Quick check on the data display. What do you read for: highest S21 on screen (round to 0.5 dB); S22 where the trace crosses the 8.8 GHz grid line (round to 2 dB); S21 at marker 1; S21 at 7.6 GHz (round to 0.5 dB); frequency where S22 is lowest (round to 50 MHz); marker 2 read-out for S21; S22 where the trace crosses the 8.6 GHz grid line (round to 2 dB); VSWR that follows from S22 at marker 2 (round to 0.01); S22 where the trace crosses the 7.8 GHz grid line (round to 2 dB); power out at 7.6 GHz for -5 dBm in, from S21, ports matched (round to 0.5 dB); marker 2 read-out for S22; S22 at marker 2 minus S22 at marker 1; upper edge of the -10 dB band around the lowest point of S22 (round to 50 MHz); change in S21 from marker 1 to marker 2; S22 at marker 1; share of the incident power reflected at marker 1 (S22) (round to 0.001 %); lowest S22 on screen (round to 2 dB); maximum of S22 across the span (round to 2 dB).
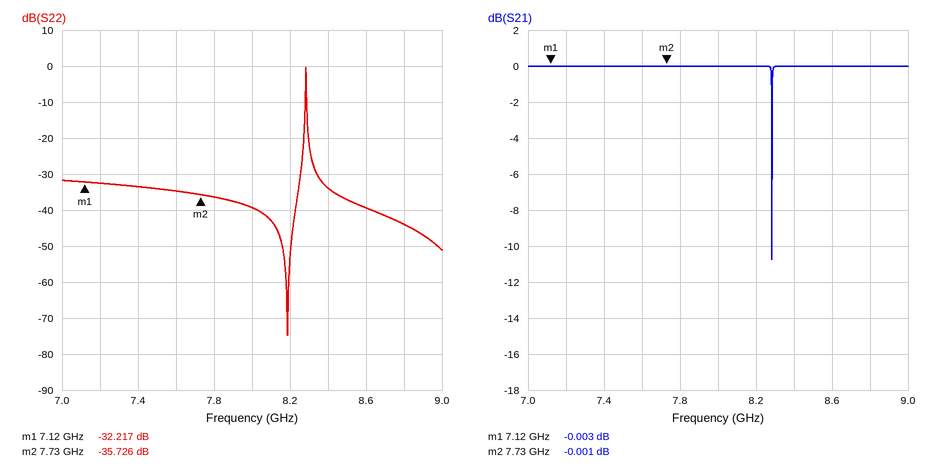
0.0 dB
-44 dB
-0.003 dB
0.0 dB
8.20 GHz
-0.001 dB
-40 dB
1.03
-36 dB
-5.0 dBm
-35.726 dB
-3.509 dB
8.30 GHz
0.002 dB
-32.217 dB
0.060 %
-74 dB
0 dB
